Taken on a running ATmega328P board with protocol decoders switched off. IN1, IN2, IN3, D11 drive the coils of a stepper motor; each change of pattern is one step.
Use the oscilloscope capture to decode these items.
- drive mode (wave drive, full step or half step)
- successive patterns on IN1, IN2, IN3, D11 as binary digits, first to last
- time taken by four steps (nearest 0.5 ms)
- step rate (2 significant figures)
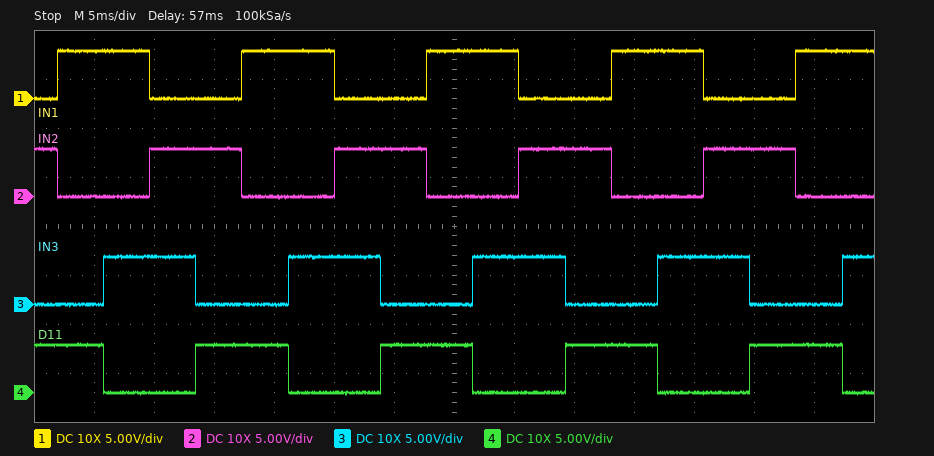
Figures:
full step
0101 1001 1010 0110 0101 1001 1010 0110 0101 1001 1010 0110 0101 1001 1010 0110 0101 1001 1010
15.5 ms
260 steps/s
